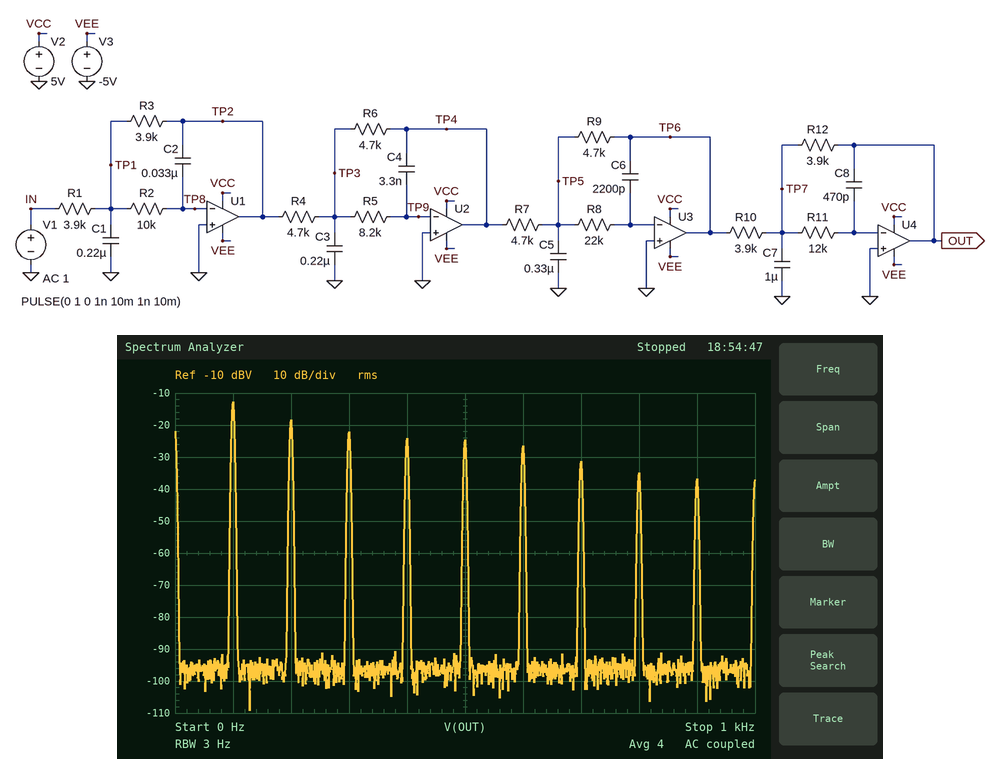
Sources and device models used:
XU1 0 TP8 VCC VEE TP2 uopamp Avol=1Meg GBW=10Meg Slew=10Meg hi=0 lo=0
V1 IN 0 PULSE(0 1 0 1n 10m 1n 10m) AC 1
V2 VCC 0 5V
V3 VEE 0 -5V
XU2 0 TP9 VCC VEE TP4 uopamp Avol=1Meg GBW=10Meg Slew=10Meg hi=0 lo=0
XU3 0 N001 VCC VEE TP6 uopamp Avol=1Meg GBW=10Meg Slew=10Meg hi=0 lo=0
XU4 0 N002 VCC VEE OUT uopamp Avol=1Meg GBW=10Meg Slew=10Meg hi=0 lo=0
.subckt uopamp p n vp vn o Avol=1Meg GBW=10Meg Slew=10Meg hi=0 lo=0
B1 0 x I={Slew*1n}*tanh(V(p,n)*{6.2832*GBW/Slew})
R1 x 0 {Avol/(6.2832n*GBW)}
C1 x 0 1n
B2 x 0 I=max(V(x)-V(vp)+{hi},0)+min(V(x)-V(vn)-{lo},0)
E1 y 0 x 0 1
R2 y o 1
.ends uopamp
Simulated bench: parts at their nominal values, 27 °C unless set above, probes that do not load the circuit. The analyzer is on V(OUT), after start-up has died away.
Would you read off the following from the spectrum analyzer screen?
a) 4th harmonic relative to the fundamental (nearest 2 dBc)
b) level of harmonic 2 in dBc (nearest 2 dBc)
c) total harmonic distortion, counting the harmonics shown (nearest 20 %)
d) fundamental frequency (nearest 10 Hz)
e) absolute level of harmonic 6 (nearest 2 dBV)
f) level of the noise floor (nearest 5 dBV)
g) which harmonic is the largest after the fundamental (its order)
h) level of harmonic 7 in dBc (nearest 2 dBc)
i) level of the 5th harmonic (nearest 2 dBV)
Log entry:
-12 dBc
-6 dBc
80 %
100 Hz
-26 dBV
-95 dBV
2
-18 dBc
-24 dBV
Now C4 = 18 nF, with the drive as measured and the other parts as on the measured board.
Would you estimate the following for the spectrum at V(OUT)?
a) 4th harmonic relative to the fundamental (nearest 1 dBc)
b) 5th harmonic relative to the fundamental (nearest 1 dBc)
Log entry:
-13 dBc
-17 dBc
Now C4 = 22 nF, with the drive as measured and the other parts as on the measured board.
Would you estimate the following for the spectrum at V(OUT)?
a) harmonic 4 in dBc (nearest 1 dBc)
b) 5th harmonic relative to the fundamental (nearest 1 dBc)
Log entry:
-15 dBc
-19 dBc
